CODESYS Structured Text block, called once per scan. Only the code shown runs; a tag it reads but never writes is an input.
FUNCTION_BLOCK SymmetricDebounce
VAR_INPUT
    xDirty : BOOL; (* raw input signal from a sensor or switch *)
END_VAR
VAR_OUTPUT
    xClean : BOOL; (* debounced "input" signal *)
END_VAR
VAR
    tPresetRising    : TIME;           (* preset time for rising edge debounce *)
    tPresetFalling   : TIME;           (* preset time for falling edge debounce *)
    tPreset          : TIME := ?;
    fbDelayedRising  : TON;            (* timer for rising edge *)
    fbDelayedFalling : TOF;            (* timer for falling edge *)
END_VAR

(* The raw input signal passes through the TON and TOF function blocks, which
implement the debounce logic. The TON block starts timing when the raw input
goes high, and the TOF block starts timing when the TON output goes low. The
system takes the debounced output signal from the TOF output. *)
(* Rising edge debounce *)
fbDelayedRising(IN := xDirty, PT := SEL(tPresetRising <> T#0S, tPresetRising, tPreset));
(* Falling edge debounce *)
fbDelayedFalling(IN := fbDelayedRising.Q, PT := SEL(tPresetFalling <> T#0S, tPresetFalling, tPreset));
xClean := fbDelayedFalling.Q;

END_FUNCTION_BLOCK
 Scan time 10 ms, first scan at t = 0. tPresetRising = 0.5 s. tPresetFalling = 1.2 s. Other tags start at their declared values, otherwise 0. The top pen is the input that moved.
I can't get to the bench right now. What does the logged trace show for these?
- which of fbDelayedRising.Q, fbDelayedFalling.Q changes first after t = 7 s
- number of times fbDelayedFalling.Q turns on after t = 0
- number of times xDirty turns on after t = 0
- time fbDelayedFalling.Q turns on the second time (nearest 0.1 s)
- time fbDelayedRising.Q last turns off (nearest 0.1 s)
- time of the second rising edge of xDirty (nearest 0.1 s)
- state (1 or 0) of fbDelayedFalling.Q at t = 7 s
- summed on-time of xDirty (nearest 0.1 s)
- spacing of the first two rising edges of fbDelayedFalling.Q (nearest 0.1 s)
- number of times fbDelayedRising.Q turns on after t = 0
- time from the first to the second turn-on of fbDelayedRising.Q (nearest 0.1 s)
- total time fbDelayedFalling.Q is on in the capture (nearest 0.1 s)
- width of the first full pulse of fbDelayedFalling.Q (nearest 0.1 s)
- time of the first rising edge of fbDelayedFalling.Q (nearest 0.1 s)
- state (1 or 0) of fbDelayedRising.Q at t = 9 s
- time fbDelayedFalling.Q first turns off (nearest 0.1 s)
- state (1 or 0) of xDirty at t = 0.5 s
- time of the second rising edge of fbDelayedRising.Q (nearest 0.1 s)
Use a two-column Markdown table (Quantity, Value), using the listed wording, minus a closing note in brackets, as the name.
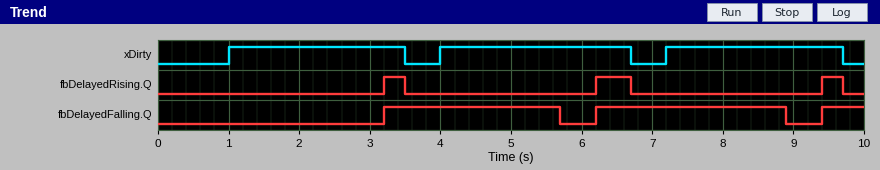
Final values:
| Quantity | Value |
|---|---|
| which of fbDelayedRising.Q, fbDelayedFalling.Q changes first after t = 7 s | fbDelayedFalling.Q |
| number of times fbDelayedFalling.Q turns on after t = 0 | 3 |
| number of times xDirty turns on after t = 0 | 3 |
| time fbDelayedFalling.Q turns on the second time | 6.2 s |
| time fbDelayedRising.Q last turns off | 9.7 s |
| time of the second rising edge of xDirty | 4.0 s |
| state (1 or 0) of fbDelayedFalling.Q at t = 7 s | 1 |
| summed on-time of xDirty | 7.7 s |
| spacing of the first two rising edges of fbDelayedFalling.Q | 3.0 s |
| number of times fbDelayedRising.Q turns on after t = 0 | 3 |
| time from the first to the second turn-on of fbDelayedRising.Q | 3.0 s |
| total time fbDelayedFalling.Q is on in the capture | 5.8 s |
| width of the first full pulse of fbDelayedFalling.Q | 2.5 s |
| time of the first rising edge of fbDelayedFalling.Q | 3.2 s |
| state (1 or 0) of fbDelayedRising.Q at t = 9 s | 0 |
| time fbDelayedFalling.Q first turns off | 5.7 s |
| state (1 or 0) of xDirty at t = 0.5 s | 0 |
| time of the second rising edge of fbDelayedRising.Q | 6.2 s |
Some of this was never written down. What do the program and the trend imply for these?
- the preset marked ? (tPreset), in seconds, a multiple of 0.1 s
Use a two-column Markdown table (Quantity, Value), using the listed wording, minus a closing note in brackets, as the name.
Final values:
| Quantity | Value |
|---|---|
| the preset marked ? (tPreset), in seconds, a multiple of 0.1 s | 2.2 s |
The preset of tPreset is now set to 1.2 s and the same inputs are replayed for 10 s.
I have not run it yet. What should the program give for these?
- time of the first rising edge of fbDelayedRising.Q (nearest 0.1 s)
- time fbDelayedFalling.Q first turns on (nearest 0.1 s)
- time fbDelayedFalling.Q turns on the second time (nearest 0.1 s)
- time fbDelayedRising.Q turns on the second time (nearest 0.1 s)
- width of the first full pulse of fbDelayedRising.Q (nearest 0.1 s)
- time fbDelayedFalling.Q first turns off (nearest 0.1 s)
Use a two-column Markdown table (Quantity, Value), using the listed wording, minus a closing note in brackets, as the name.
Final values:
| Quantity | Value |
|---|---|
| time of the first rising edge of fbDelayedRising.Q | 2.2 s |
| time fbDelayedFalling.Q first turns on | 2.2 s |
| time fbDelayedFalling.Q turns on the second time | 5.2 s |
| time fbDelayedRising.Q turns on the second time | 5.2 s |
| width of the first full pulse of fbDelayedRising.Q | 1.3 s |
| time fbDelayedFalling.Q first turns off | 4.7 s |
